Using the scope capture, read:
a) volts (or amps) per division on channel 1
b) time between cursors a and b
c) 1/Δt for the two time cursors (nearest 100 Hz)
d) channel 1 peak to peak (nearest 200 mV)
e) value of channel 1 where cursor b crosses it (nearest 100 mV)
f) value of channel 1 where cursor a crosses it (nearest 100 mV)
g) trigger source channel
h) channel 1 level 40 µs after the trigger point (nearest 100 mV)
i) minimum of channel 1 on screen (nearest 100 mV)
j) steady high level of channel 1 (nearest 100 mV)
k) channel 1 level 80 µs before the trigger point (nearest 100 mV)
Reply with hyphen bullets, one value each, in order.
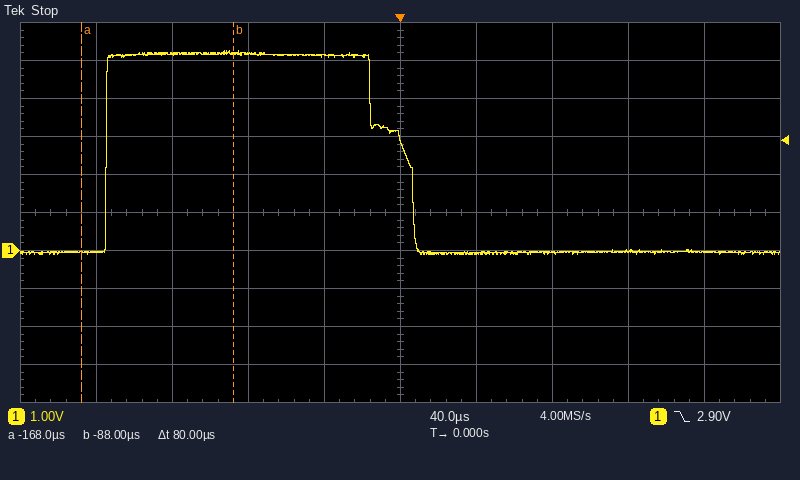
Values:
- 1 V
- 80 µs
- 12.5 kHz
- 5.4 V
- 5.2 V
- 0.0 V
- channel 1
- -100 mV
- -100 mV
- 5.2 V
- 5.2 V
